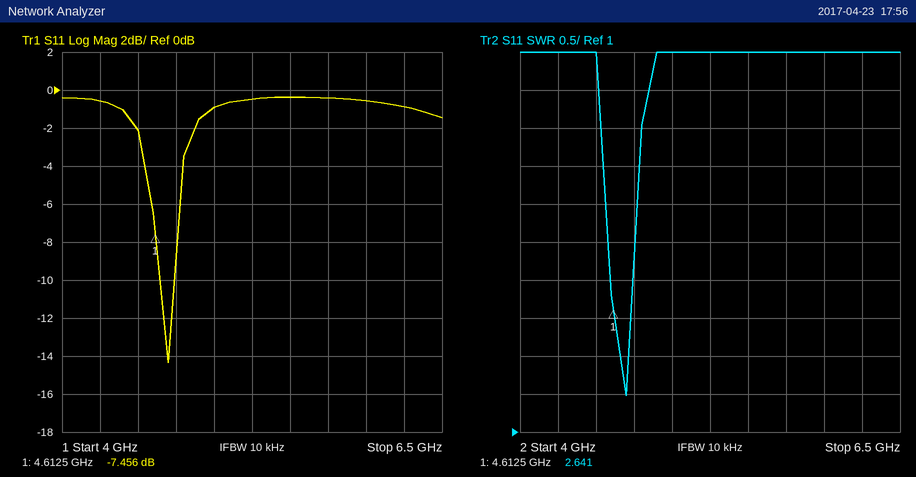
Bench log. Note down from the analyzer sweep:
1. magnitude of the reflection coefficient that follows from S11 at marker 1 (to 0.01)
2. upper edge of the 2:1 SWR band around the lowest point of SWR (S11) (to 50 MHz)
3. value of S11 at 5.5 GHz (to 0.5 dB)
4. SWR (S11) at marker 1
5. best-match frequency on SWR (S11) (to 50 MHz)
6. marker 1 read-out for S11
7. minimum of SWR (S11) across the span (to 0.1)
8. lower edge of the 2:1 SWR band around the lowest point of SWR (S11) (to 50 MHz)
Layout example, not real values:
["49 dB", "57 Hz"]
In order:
["0.42", "4.70 GHz", "-0.5 dB", "2.641", "4.70 GHz", "-7.456 dB", "1.5", "4.65 GHz"]
